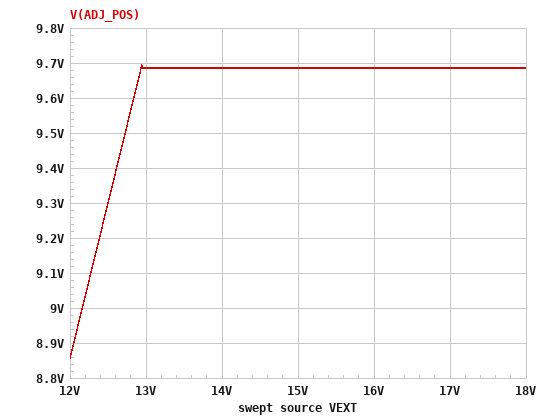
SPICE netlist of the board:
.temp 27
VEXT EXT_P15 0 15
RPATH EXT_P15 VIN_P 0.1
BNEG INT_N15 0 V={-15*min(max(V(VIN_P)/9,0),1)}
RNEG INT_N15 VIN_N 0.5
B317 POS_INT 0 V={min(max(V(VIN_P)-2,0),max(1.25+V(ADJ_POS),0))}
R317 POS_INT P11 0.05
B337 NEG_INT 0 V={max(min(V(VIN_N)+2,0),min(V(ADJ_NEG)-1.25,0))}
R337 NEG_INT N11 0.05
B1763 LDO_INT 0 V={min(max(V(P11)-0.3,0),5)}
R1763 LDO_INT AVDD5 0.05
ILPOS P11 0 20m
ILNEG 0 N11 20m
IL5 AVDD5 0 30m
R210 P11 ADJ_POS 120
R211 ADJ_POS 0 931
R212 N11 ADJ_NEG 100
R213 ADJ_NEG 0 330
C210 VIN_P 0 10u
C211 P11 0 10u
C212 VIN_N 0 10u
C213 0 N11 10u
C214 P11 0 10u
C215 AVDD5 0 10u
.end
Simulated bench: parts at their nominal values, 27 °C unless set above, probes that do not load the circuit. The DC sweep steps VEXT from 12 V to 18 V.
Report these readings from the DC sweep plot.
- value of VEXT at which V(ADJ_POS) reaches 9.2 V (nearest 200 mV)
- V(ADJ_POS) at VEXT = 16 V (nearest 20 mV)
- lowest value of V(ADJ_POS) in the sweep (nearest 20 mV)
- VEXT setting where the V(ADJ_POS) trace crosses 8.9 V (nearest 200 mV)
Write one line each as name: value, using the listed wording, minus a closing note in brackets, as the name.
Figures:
value of VEXT at which V(ADJ_POS) reaches 9.2 V: 12.4 V
V(ADJ_POS) at VEXT = 16 V: 9.68 V
lowest value of V(ADJ_POS) in the sweep: 8.86 V
VEXT setting where the V(ADJ_POS) trace crosses 8.9 V: 12.0 V
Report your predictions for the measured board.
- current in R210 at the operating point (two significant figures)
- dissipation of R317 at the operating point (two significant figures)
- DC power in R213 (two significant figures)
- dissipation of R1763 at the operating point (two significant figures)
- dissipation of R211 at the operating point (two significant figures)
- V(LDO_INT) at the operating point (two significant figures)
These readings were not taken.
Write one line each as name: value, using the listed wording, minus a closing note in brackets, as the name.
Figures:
current in R210 at the operating point: 10 mA
dissipation of R317 at the operating point: 46 µW
DC power in R213: 51 mW
dissipation of R1763 at the operating point: 45 µW
dissipation of R211 at the operating point: 100 mW
V(LDO_INT) at the operating point: 5.0 V
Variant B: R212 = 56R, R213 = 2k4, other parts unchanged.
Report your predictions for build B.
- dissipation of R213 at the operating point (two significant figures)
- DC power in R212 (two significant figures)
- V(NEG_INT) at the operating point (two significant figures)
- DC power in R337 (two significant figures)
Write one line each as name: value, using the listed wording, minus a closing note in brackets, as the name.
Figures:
dissipation of R213 at the operating point: 67 mW
DC power in R212: 1.6 mW
V(NEG_INT) at the operating point: -13 V
DC power in R337: 32 µW
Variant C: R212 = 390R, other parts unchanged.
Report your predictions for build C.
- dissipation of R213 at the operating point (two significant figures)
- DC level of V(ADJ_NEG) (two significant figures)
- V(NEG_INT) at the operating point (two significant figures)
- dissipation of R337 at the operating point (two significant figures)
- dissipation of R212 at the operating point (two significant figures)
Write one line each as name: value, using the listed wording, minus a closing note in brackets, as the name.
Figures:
dissipation of R213 at the operating point: 3.4 mW
DC level of V(ADJ_NEG): -1.1 V
V(NEG_INT) at the operating point: -2.3 V
dissipation of R337 at the operating point: 27 µW
dissipation of R212 at the operating point: 4.0 mW
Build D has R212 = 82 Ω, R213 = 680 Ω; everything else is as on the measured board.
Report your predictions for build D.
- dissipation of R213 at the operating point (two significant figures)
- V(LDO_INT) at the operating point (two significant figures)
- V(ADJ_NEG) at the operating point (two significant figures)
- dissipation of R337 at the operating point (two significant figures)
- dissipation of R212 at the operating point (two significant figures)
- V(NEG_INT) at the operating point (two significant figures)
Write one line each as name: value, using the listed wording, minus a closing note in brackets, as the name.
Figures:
dissipation of R213 at the operating point: 160 mW
V(LDO_INT) at the operating point: 5.0 V
V(ADJ_NEG) at the operating point: -10 V
dissipation of R337 at the operating point: 62 µW
dissipation of R212 at the operating point: 19 mW
V(NEG_INT) at the operating point: -12 V
